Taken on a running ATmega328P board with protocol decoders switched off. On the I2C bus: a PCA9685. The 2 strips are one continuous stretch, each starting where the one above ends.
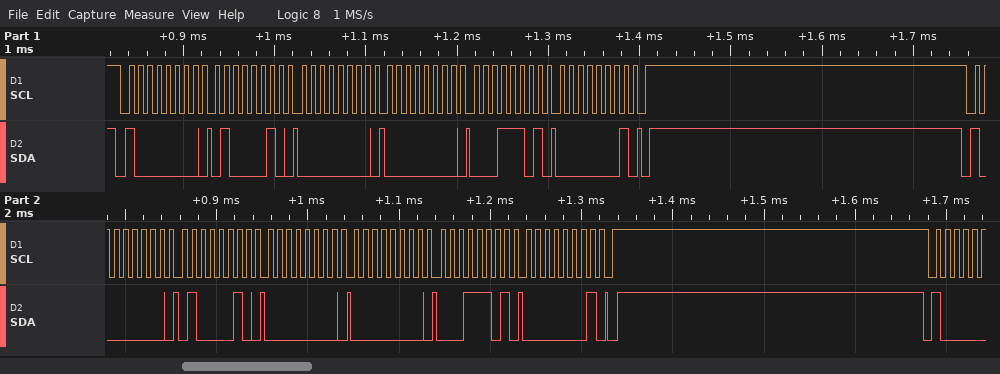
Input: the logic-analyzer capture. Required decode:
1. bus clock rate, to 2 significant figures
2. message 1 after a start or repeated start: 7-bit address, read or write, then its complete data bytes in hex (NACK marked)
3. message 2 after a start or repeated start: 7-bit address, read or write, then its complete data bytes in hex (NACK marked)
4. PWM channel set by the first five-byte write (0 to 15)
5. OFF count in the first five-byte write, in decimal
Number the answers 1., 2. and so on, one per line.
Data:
1. 100 kHz
2. 0x40 write: 42 00 00 1D 01
3. 0x40 write: 42 00 00 1D 01
4. 15
5. 285
